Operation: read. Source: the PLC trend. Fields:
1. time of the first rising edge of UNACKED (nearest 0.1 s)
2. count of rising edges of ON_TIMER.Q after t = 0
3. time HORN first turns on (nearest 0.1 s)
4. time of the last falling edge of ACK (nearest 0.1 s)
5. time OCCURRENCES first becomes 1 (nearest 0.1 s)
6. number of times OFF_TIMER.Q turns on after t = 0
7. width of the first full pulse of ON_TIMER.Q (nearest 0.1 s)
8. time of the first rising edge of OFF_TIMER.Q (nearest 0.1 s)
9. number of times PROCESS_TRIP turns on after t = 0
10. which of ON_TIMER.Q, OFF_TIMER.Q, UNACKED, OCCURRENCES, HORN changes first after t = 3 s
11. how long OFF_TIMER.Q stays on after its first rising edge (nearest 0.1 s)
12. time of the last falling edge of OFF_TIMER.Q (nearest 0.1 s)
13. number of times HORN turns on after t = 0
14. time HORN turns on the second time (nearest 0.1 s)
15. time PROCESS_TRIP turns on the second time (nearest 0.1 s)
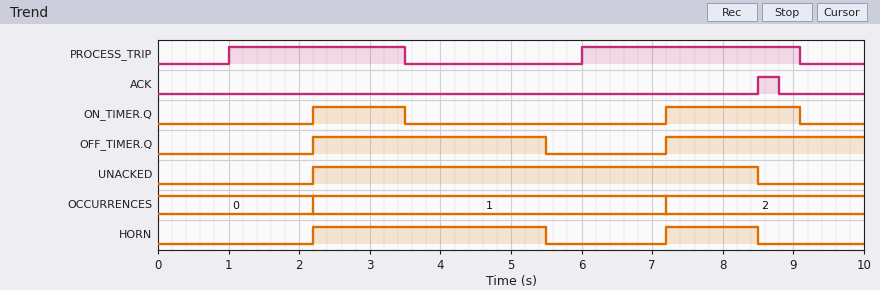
2.2 s
2
2.2 s
8.8 s
2.2 s
2
1.3 s
2.2 s
2
ON_TIMER.Q
3.3 s
5.5 s
2
7.2 s
6.0 s
